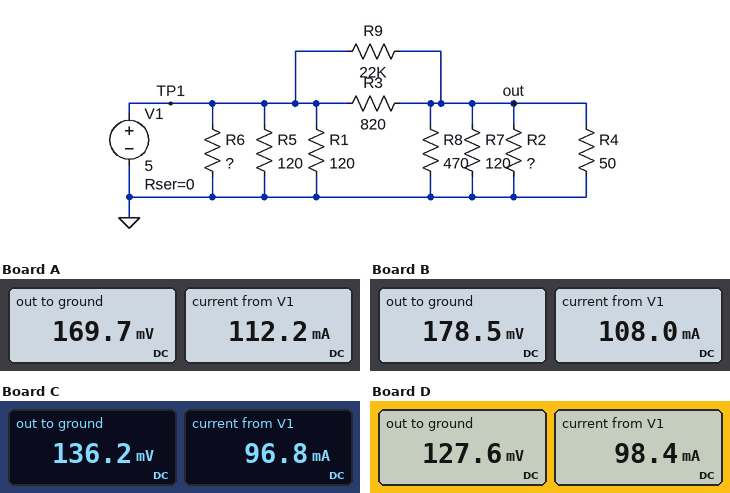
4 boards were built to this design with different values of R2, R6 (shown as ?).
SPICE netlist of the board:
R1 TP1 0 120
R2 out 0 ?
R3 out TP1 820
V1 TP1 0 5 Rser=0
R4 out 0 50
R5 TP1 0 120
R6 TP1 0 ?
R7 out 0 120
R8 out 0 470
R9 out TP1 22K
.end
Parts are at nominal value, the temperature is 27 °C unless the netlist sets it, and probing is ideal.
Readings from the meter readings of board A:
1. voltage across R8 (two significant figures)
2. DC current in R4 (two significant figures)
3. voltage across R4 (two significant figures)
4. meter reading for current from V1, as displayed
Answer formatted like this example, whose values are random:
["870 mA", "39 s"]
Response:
["170 mV", "3.4 mA", "170 mV", "112.2 mA"]
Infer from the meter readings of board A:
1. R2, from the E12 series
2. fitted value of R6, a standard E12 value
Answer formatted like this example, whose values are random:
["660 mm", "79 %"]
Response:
["180 Ω", "220 Ω"]
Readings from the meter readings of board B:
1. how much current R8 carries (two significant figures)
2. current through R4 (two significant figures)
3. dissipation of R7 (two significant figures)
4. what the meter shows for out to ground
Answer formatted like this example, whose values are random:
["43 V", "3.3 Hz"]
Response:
["380 µA", "3.6 mA", "270 µW", "178.5 mV"]
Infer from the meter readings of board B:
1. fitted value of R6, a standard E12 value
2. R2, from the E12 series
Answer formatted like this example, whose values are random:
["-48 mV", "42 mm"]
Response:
["270 Ω", "270 Ω"]
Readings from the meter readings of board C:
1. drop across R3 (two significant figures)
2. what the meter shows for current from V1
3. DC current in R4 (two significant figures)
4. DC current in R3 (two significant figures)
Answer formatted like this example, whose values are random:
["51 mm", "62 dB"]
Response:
["4.9 V", "96.8 mA", "2.7 mA", "5.9 mA"]
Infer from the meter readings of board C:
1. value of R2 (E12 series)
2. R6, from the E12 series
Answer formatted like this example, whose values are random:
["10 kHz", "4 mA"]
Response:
["68 Ω", "680 Ω"]
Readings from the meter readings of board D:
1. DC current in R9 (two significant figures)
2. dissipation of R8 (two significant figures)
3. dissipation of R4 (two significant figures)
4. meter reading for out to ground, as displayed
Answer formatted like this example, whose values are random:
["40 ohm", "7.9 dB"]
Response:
["220 µA", "35 µW", "330 µW", "127.6 mV"]
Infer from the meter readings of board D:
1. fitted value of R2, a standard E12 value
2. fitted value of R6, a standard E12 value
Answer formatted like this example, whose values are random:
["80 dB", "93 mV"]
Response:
["56 Ω", "560 Ω"]
